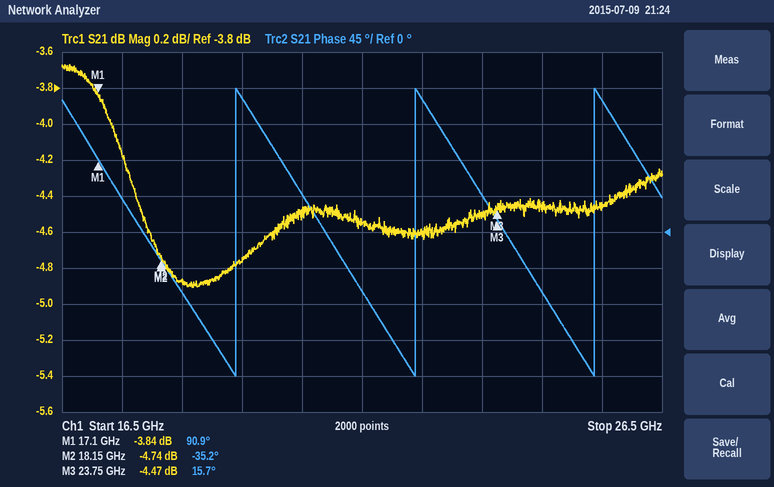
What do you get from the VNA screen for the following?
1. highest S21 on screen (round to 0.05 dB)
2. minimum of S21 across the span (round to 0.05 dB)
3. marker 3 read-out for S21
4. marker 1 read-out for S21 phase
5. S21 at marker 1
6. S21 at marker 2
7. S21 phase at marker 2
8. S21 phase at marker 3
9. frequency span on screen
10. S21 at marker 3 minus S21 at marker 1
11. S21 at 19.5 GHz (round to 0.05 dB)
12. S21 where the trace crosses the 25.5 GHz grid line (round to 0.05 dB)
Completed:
-3.65 dB
-4.90 dB
-4.47 dB
90.9°
-3.84 dB
-4.74 dB
-35.2°
15.7°
10 GHz
-0.63 dB
-4.75 dB
-4.45 dB
